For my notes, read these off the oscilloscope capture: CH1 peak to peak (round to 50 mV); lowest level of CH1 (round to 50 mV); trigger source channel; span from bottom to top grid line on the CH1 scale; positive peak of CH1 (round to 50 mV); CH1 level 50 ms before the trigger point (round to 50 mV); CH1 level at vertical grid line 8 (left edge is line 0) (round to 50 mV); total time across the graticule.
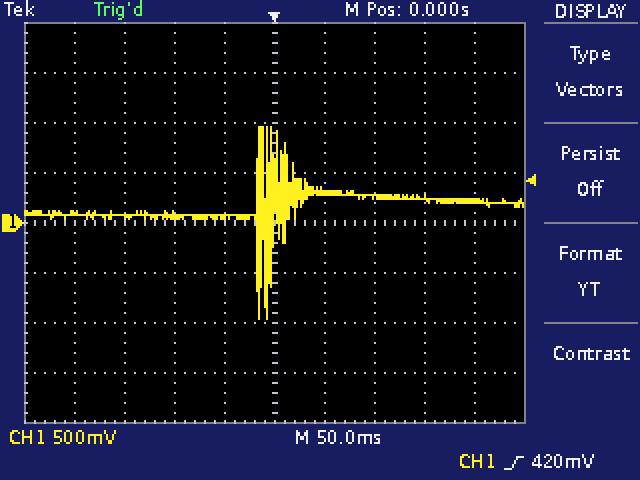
1.90 V
-950 mV
CH1
4 V
950 mV
50 mV
250 mV
500 ms
